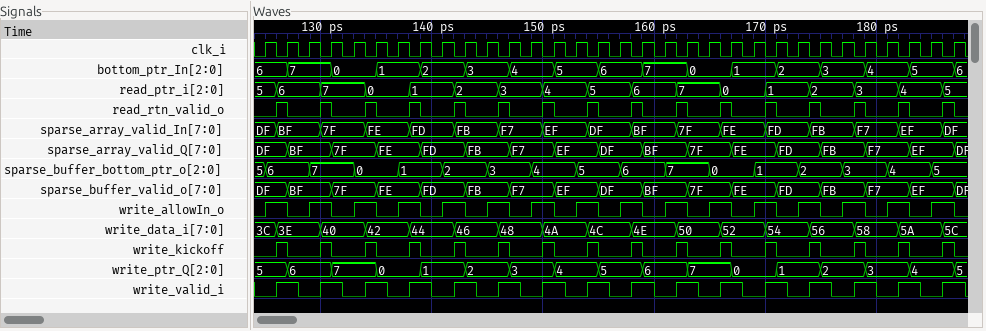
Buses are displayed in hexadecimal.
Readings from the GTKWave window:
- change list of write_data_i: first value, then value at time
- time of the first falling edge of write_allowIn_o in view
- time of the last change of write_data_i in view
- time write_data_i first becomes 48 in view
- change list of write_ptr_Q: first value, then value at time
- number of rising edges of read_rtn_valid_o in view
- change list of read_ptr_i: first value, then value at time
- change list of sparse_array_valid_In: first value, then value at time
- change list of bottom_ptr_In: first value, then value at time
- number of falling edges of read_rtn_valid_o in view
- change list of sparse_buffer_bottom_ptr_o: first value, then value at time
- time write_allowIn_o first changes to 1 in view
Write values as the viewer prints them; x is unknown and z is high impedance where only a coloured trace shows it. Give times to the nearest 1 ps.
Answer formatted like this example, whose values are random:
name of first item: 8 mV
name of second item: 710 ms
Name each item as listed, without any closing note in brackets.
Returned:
change list of write_data_i: first value, then value at time: 3C, 3E at 126 ps, 40 at 130 ps, 42 at 134 ps, 44 at 138 ps, 46 at 142 ps, 48 at 146 ps, 4A at 150 ps, 4C at 154 ps, 4E at 158 ps, 50 at 162 ps, 52 at 166 ps, 54 at 170 ps, 56 at 174 ps, 58 at 178 ps, 5A at 182 ps, 5C at 186 ps
time of the first falling edge of write_allowIn_o in view: 127 ps
time of the last change of write_data_i in view: 186 ps
time write_data_i first becomes 48 in view: 146 ps
change list of write_ptr_Q: first value, then value at time: 5, 6 at 127 ps, 7 at 131 ps, 0 at 135 ps, 1 at 139 ps, 2 at 143 ps, 3 at 147 ps, 4 at 151 ps, 5 at 155 ps, 6 at 159 ps, 7 at 163 ps, 0 at 167 ps, 1 at 171 ps, 2 at 175 ps, 3 at 179 ps, 4 at 183 ps, 5 at 187 ps
number of rising edges of read_rtn_valid_o in view: 16
change list of read_ptr_i: first value, then value at time: 5, 6 at 126 ps, 7 at 130 ps, 0 at 134 ps, 1 at 138 ps, 2 at 142 ps, 3 at 146 ps, 4 at 150 ps, 5 at 154 ps, 6 at 158 ps, 7 at 162 ps, 0 at 166 ps, 1 at 170 ps, 2 at 174 ps, 3 at 178 ps, 4 at 182 ps, 5 at 186 ps
change list of sparse_array_valid_In: first value, then value at time: DF, BF at 126 ps, 7F at 130 ps, FE at 134 ps, FD at 138 ps, FB at 142 ps, F7 at 146 ps, EF at 150 ps, DF at 154 ps, BF at 158 ps, 7F at 162 ps, FE at 166 ps, FD at 170 ps, FB at 174 ps, F7 at 178 ps, EF at 182 ps, DF at 186 ps
change list of bottom_ptr_In: first value, then value at time: 6, 7 at 127 ps, 0 at 131 ps, 1 at 135 ps, 2 at 139 ps, 3 at 143 ps, 4 at 147 ps, 5 at 151 ps, 6 at 155 ps, 7 at 159 ps, 0 at 163 ps, 1 at 167 ps, 2 at 171 ps, 3 at 175 ps, 4 at 179 ps, 5 at 183 ps, 6 at 187 ps
number of falling edges of read_rtn_valid_o in view: 16
change list of sparse_buffer_bottom_ptr_o: first value, then value at time: 5, 6 at 125 ps, 7 at 129 ps, 0 at 133 ps, 1 at 137 ps, 2 at 141 ps, 3 at 145 ps, 4 at 149 ps, 5 at 153 ps, 6 at 157 ps, 7 at 161 ps, 0 at 165 ps, 1 at 169 ps, 2 at 173 ps, 3 at 177 ps, 4 at 181 ps, 5 at 185 ps
time write_allowIn_o first changes to 1 in view: 125 ps
